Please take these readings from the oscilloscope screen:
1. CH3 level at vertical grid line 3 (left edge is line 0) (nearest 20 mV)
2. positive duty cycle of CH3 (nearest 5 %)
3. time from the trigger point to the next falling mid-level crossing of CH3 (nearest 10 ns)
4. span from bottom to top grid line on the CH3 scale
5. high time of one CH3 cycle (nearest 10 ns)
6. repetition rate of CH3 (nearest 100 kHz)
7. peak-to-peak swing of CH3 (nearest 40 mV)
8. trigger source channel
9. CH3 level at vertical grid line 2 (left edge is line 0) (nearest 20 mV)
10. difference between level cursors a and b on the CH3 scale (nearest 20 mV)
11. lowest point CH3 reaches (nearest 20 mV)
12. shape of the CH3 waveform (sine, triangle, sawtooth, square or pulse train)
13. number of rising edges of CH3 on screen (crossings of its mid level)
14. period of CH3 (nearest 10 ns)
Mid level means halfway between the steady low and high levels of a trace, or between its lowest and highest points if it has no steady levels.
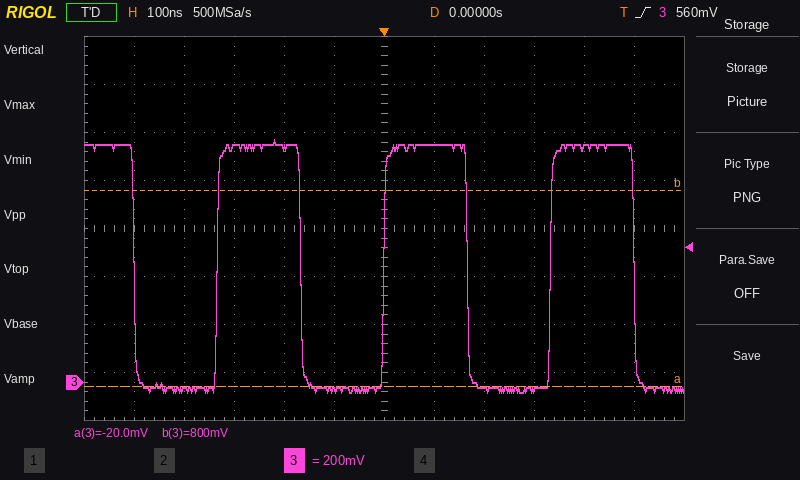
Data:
980 mV
50 %
170 ns
1.6 V
170 ns
3.0 MHz
1.04 V
CH3
-40 mV
820 mV
-40 mV
square
3
330 ns
